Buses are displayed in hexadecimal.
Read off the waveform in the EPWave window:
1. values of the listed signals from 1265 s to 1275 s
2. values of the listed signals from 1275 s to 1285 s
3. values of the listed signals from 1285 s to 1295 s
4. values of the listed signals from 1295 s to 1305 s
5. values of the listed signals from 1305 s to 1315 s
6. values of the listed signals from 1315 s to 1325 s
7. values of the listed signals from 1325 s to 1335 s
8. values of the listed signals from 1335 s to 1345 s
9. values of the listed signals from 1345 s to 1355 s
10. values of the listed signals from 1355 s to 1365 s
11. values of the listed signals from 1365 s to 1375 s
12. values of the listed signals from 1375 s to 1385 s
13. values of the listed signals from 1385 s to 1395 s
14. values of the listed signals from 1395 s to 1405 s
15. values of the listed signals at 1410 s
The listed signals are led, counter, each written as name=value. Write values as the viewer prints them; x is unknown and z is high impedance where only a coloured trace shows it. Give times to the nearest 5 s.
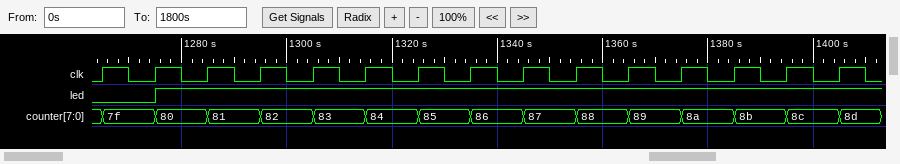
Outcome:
led=0, counter=7f
led=1, counter=80
led=1, counter=81
led=1, counter=82
led=1, counter=83
led=1, counter=84
led=1, counter=85
led=1, counter=86
led=1, counter=87
led=1, counter=88
led=1, counter=89
led=1, counter=8a
led=1, counter=8b
led=1, counter=8c
led=1, counter=8d
